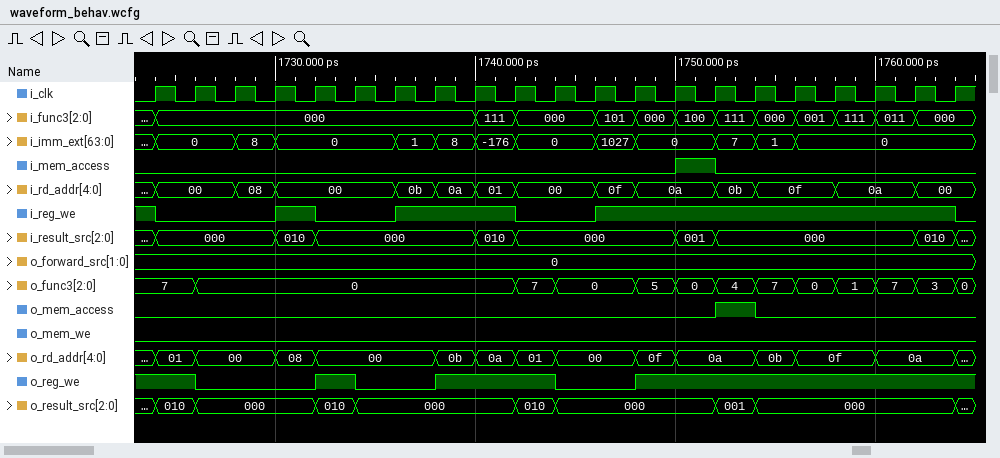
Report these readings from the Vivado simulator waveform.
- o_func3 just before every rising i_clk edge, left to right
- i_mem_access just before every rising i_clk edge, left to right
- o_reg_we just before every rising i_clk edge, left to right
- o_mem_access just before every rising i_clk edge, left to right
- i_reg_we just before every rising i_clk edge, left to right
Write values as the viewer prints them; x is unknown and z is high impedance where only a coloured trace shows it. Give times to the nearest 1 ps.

7, 7, 0, 0, 0, 0, 0, 0, 0, 0, 7, 0, 0, 5, 0, 4, 7, 0, 1, 7, 3
0 0 0 0 0 0 0 0 0 0 0 0 0 0 1 0 0 0 0 0 0
1 1 0 0 0 1 0 0 1 1 1 0 0 1 1 1 1 1 1 1 1
0 0 0 0 0 0 0 0 0 0 0 0 0 0 0 1 0 0 0 0 0
1 0 0 0 1 0 0 1 1 1 0 0 1 1 1 1 1 1 1 1 1
